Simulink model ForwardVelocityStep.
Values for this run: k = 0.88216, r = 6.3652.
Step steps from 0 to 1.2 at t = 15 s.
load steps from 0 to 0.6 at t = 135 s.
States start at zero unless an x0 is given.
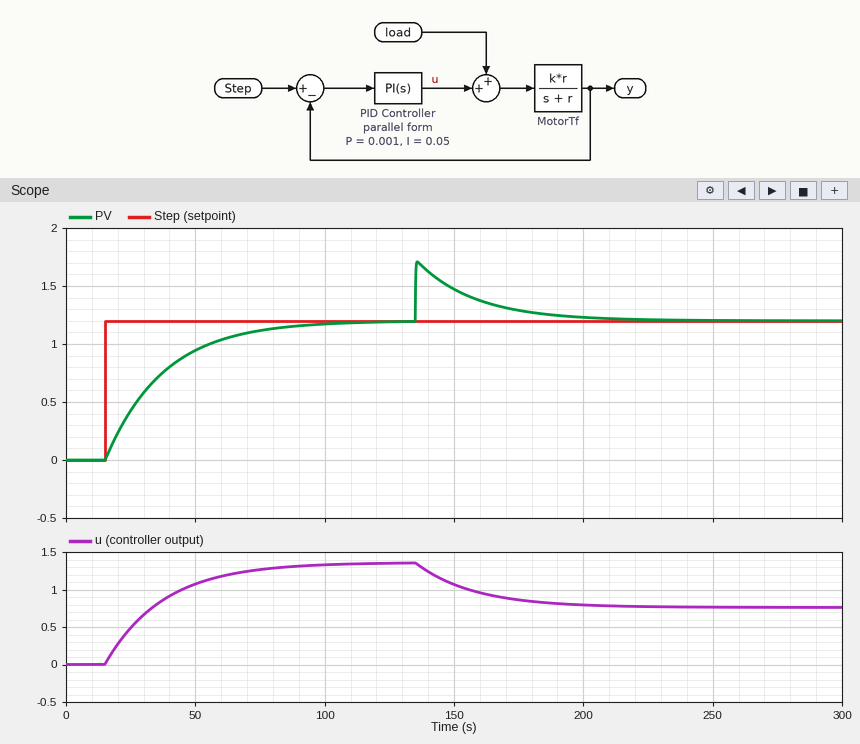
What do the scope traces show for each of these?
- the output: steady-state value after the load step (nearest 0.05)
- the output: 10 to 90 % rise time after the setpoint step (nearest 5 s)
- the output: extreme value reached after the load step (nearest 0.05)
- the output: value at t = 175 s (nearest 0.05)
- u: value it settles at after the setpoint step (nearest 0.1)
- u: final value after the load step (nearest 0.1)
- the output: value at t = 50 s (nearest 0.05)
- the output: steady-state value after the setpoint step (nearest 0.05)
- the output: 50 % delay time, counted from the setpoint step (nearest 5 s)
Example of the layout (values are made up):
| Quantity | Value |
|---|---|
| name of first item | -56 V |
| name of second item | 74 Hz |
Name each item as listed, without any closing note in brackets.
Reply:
| Quantity | Value |
|---|---|
| the output: steady-state value after the load step | 1.20 |
| the output: 10 to 90 % rise time after the setpoint step | 50 s |
| the output: extreme value reached after the load step | 1.70 |
| the output: value at t = 175 s | 1.30 |
| u: value it settles at after the setpoint step | 1.4 |
| u: final value after the load step | 0.8 |
| the output: value at t = 50 s | 0.95 |
| the output: steady-state value after the setpoint step | 1.20 |
| the output: 50 % delay time, counted from the setpoint step | 15 s |
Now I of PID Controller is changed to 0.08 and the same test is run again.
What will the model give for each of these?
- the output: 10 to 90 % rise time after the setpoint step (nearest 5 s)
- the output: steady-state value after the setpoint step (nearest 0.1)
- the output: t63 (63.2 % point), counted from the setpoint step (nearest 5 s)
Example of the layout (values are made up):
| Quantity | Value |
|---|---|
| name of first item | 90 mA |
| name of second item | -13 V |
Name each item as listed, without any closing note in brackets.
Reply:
| Quantity | Value |
|---|---|
| the output: 10 to 90 % rise time after the setpoint step | 30 s |
| the output: steady-state value after the setpoint step | 1.2 |
| the output: t63 (63.2 % point), counted from the setpoint step | 15 s |
